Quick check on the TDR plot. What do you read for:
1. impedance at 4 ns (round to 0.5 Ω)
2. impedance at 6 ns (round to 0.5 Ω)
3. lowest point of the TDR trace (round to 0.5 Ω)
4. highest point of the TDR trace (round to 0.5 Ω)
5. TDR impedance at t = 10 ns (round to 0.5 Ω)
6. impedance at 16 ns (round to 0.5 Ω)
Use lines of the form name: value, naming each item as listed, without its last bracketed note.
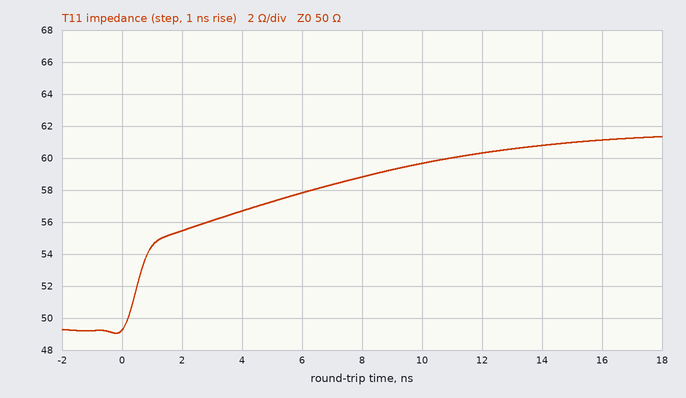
impedance at 4 ns: 56.5 Ω
impedance at 6 ns: 58.0 Ω
lowest point of the TDR trace: 49.0 Ω
highest point of the TDR trace: 61.5 Ω
TDR impedance at t = 10 ns: 59.5 Ω
impedance at 16 ns: 61.0 Ω
